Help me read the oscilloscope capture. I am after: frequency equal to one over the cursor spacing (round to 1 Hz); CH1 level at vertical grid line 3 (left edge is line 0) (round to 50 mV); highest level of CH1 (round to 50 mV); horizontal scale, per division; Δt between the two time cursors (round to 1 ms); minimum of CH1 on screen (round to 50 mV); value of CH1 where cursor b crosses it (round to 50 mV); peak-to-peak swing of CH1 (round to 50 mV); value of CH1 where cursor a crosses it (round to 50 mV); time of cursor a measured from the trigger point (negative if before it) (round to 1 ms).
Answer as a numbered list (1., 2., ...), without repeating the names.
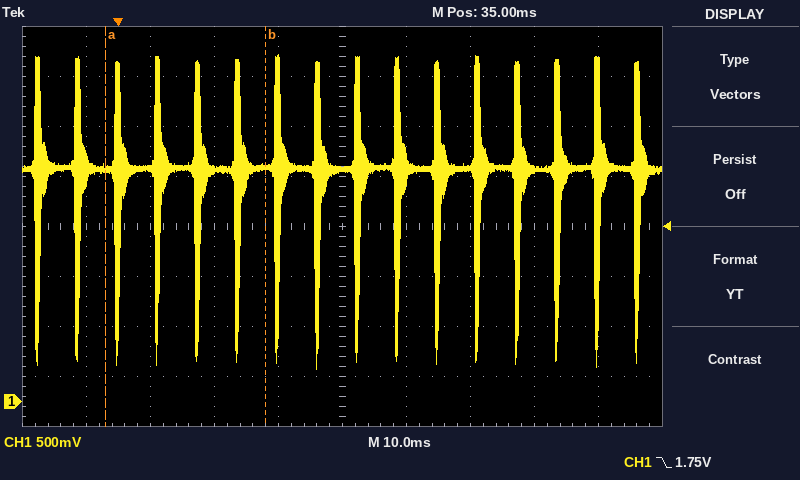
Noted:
1. 40 Hz
2. 2.30 V
3. 3.45 V
4. 10 ms
5. 25 ms
6. 300 mV
7. 2.35 V
8. 3.15 V
9. 2.35 V
10. -2 ms
